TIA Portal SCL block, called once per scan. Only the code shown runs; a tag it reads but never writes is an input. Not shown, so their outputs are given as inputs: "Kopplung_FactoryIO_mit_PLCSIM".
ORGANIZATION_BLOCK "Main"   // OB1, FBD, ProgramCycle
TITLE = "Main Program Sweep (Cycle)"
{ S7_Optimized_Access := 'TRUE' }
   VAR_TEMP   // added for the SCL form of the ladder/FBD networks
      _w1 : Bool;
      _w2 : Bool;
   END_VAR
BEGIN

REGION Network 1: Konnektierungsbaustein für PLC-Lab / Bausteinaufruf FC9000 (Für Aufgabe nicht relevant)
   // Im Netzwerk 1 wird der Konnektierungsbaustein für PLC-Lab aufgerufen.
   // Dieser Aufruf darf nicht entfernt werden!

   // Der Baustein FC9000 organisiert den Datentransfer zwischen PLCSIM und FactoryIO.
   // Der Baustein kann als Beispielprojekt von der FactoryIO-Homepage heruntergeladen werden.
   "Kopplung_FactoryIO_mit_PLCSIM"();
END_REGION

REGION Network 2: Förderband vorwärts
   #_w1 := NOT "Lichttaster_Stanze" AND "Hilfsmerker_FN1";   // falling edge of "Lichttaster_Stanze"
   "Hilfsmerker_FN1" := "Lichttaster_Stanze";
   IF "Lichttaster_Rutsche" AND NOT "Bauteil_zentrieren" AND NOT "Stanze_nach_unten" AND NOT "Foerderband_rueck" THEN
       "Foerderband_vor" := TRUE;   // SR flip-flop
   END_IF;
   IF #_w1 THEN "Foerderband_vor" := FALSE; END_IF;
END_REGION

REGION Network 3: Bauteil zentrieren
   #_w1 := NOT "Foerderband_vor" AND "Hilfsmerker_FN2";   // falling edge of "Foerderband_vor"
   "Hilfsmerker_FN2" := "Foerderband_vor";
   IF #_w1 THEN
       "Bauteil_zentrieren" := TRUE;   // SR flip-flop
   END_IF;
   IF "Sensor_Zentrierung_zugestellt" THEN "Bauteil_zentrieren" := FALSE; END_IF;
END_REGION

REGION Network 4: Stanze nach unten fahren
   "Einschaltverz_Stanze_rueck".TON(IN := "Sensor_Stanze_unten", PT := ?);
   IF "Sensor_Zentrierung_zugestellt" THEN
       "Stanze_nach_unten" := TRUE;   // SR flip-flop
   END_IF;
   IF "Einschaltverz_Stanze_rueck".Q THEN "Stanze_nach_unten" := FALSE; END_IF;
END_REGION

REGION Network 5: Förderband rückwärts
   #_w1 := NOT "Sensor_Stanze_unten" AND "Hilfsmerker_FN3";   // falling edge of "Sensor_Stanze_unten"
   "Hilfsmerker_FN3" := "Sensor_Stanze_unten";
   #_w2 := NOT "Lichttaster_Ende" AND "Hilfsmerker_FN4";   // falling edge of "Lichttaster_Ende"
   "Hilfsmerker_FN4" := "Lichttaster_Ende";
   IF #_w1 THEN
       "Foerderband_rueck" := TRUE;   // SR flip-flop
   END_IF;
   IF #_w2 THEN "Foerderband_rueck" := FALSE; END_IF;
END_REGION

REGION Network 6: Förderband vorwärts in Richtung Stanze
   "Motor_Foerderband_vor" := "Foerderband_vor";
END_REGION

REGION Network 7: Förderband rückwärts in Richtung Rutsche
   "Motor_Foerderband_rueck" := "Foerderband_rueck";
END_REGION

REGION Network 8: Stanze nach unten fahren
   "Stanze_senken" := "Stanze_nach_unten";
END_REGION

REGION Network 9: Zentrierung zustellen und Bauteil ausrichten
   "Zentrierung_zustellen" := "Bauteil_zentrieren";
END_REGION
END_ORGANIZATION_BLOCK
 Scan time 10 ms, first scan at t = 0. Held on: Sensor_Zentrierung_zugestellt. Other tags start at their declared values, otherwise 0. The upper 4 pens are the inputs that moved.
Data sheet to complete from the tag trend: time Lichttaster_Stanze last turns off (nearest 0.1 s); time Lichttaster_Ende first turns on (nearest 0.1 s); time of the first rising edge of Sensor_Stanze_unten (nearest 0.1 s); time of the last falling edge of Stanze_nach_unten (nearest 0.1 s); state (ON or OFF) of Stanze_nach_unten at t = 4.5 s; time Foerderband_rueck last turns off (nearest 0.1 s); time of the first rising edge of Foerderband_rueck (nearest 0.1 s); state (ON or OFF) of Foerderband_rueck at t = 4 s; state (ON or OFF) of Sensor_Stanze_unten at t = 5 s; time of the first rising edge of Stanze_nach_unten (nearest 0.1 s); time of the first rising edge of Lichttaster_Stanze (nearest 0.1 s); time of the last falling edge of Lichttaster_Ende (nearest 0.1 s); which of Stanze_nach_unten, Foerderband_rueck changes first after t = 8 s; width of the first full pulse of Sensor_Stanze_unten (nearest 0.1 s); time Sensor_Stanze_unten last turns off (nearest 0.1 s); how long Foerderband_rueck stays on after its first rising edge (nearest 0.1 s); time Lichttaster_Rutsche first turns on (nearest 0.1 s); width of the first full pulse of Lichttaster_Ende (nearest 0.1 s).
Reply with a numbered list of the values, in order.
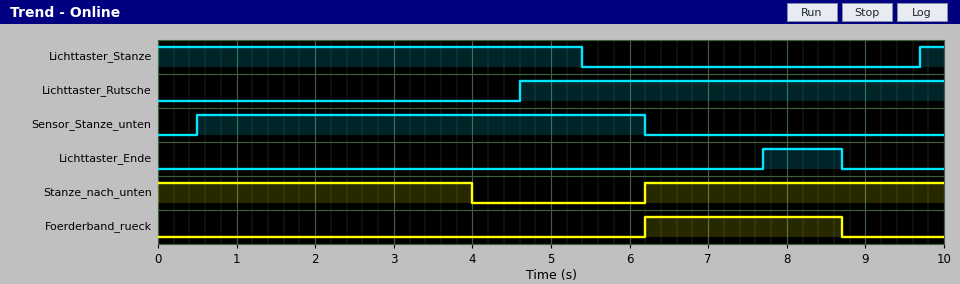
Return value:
1. 5.4 s
2. 7.7 s
3. 0.5 s
4. 4.0 s
5. OFF
6. 8.7 s
7. 6.2 s
8. OFF
9. ON
10. 6.2 s
11. 9.7 s
12. 8.7 s
13. Foerderband_rueck
14. 5.7 s
15. 6.2 s
16. 2.5 s
17. 4.6 s
18. 1.0 s
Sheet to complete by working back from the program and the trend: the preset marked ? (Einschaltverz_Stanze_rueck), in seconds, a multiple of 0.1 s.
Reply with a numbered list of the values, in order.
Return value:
1. 3.5 s
